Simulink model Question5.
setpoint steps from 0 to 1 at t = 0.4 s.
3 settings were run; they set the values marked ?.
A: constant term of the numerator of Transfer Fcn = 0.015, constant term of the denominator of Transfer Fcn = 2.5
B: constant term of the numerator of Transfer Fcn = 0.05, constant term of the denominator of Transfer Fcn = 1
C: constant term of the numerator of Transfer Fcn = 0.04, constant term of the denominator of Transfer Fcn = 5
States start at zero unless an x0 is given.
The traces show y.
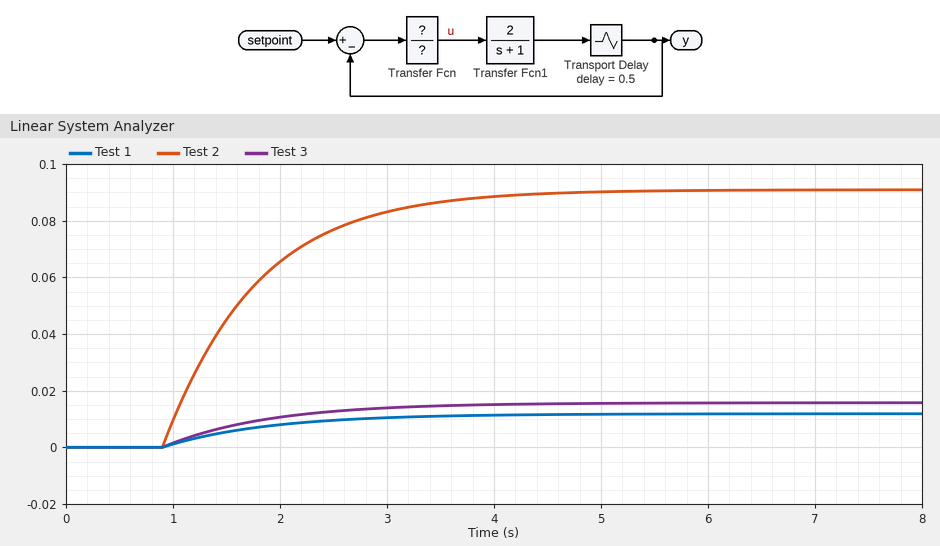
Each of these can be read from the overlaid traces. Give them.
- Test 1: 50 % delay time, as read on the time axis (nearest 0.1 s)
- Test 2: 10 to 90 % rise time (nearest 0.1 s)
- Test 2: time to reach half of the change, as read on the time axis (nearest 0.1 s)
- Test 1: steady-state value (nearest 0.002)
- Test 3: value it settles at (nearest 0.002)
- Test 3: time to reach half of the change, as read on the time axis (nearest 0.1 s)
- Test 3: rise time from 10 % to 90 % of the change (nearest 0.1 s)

1.6 s
1.9 s
1.5 s
0.012
0.016
1.6 s
2.1 s
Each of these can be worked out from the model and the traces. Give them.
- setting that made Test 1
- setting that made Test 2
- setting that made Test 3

A
B
C
